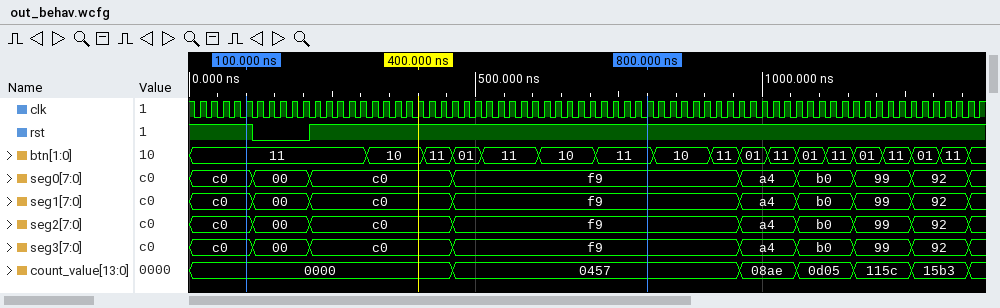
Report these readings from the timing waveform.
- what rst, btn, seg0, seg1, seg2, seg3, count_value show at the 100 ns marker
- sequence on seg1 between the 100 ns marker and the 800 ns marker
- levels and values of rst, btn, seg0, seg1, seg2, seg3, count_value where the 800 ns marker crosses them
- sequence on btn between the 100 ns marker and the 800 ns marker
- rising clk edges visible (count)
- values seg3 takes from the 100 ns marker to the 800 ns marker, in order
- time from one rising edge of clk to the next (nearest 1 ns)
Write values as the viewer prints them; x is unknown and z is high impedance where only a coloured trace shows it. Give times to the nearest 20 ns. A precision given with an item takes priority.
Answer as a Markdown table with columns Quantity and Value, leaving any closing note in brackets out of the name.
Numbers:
| Quantity | Value |
|---|---|
| what rst, btn, seg0, seg1, seg2, seg3, count_value show at the 100 ns marker | rst=1, btn=11, seg0=c0, seg1=c0, seg2=c0, seg3=c0, count_value=0000 |
| sequence on seg1 between the 100 ns marker and the 800 ns marker | c0, 00, c0, f9 |
| levels and values of rst, btn, seg0, seg1, seg2, seg3, count_value where the 800 ns marker crosses them | rst=1, btn=11, seg0=f9, seg1=f9, seg2=f9, seg3=f9, count_value=0457 |
| sequence on btn between the 100 ns marker and the 800 ns marker | 11, 10, 11, 01, 11, 10, 11 |
| rising clk edges visible | 69 |
| values seg3 takes from the 100 ns marker to the 800 ns marker, in order | c0, 00, c0, f9 |
| time from one rising edge of clk to the next | 20 ns |
